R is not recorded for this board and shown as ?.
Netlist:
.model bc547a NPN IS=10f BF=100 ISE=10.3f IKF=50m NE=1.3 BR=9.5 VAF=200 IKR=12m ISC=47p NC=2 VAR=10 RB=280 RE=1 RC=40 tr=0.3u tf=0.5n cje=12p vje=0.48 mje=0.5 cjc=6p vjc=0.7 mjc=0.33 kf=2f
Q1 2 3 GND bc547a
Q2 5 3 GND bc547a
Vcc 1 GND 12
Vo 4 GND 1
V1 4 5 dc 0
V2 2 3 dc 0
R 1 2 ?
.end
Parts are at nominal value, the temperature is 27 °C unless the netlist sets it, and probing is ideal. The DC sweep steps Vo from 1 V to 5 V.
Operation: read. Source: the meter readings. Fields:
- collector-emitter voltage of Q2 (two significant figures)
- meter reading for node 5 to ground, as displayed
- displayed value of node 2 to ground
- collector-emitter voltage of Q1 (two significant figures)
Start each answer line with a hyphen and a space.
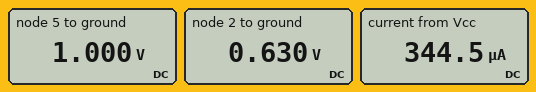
- 1.0 V
- 1.000 V
- 0.630 V
- 630 mV
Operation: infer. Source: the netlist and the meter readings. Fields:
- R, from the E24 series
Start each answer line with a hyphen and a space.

- 33 kΩ
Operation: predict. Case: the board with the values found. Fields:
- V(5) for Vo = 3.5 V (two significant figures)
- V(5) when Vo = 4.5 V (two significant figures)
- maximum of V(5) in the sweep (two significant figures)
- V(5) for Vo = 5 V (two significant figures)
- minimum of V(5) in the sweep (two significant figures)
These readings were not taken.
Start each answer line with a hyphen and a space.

- 3.5 V
- 4.5 V
- 5.0 V
- 5.0 V
- 1.0 V
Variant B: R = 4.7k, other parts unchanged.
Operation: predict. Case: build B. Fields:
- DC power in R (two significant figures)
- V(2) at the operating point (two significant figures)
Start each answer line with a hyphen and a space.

- 27 mW
- 690 mV
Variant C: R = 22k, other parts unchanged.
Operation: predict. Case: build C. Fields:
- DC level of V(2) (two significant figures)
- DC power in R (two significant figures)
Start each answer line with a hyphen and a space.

- 640 mV
- 5.9 mW
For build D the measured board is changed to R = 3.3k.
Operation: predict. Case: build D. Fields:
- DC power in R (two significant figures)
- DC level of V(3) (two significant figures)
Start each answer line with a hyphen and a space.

- 39 mW
- 710 mV
